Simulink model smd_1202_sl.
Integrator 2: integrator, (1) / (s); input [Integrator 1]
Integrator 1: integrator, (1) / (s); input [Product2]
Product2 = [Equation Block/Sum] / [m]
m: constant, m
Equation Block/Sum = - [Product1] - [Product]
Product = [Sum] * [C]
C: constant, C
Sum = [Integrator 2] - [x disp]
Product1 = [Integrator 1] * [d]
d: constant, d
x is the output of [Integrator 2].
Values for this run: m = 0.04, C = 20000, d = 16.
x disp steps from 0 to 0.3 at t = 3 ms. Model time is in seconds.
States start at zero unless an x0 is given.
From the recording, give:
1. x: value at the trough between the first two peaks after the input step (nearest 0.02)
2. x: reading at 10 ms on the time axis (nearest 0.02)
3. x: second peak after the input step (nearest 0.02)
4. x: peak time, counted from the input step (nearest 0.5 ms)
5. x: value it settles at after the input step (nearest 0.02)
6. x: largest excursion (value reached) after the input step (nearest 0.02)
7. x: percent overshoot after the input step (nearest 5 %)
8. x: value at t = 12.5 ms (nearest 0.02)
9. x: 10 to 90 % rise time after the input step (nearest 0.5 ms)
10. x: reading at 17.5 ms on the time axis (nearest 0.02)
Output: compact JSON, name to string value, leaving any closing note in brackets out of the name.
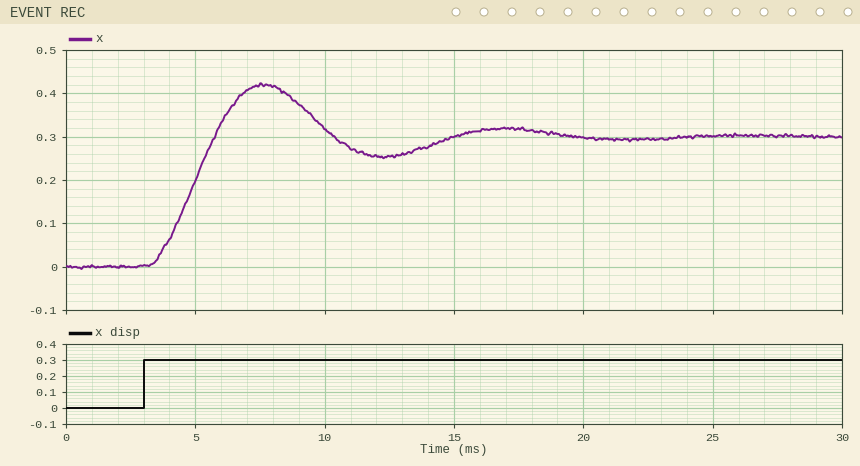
{"x: value at the trough between the first two peaks after the input step": "0.26", "x: reading at 10 ms on the time axis": "0.32", "x: second peak after the input step": "0.32", "x: peak time, counted from the input step": "4.5 ms", "x: value it settles at after the input step": "0.30", "x: largest excursion (value reached) after the input step": "0.42", "x: percent overshoot after the input step": "40 %", "x: value at t = 12.5 ms": "0.26", "x: 10 to 90 % rise time after the input step": "2.0 ms", "x: reading at 17.5 ms on the time axis": "0.32"}
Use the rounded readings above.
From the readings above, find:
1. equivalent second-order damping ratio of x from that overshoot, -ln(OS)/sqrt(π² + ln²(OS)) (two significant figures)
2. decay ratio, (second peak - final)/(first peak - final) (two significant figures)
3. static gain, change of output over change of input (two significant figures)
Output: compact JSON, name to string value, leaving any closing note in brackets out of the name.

{"equivalent second-order damping ratio of x from that overshoot, -ln(OS)/sqrt(π² + ln²(OS))": "0.28", "decay ratio, (second peak - final)/(first peak - final)": "0.17", "static gain, change of output over change of input": "1.0"}
